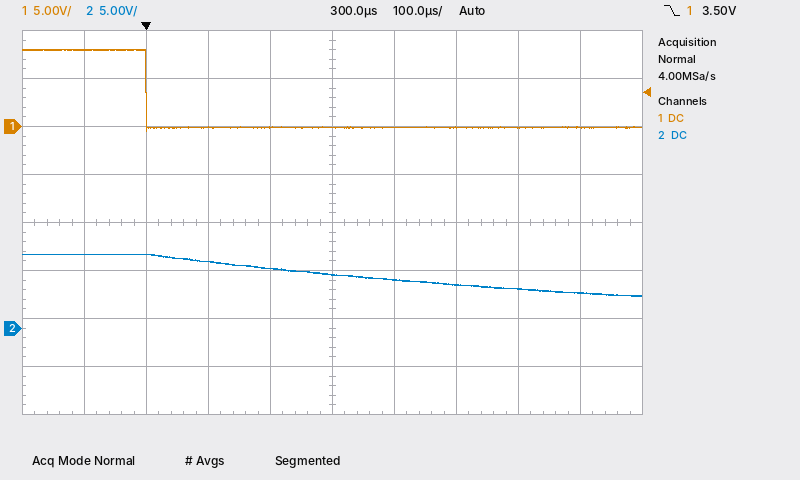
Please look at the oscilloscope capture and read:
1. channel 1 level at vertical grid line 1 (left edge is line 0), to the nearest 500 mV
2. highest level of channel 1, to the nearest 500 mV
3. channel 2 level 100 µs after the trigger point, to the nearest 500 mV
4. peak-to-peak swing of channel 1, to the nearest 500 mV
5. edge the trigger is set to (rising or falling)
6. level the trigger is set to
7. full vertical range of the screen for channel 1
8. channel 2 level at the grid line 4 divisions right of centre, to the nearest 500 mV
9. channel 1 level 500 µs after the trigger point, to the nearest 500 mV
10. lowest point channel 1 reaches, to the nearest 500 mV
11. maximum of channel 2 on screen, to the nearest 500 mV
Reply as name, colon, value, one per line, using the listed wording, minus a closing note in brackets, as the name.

channel 1 level at vertical grid line 1 (left edge is line 0), to the nearest 500 mV: 8.0 V
highest level of channel 1, to the nearest 500 mV: 8.0 V
channel 2 level 100 µs after the trigger point, to the nearest 500 mV: 7.0 V
peak-to-peak swing of channel 1, to the nearest 500 mV: 8.5 V
edge the trigger is set to: falling
level the trigger is set to: 3.50 V
full vertical range of the screen for channel 1: 40 V
channel 2 level at the grid line 4 divisions right of centre, to the nearest 500 mV: 3.5 V
channel 1 level 500 µs after the trigger point, to the nearest 500 mV: 0.0 V
lowest point channel 1 reaches, to the nearest 500 mV: -500 mV
maximum of channel 2 on screen, to the nearest 500 mV: 7.5 V
